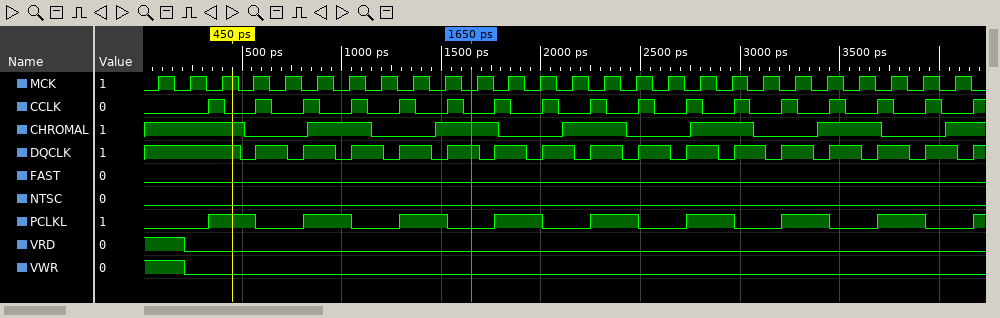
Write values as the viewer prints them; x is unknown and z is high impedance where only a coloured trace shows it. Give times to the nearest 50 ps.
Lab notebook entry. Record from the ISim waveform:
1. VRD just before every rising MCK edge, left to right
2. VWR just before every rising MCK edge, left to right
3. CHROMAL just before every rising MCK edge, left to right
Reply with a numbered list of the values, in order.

1. 1 0 0 0 0 0 0 0 0 0 0 0 0 0 0 0 0 0 0 0 0 0 0 0 0 0
2. 1 0 0 0 0 0 0 0 0 0 0 0 0 0 0 0 0 0 0 0 0 0 0 0 0 0
3. 1 1 1 0 0 1 1 0 0 1 1 0 0 1 1 0 0 1 1 0 0 1 1 0 0 1
